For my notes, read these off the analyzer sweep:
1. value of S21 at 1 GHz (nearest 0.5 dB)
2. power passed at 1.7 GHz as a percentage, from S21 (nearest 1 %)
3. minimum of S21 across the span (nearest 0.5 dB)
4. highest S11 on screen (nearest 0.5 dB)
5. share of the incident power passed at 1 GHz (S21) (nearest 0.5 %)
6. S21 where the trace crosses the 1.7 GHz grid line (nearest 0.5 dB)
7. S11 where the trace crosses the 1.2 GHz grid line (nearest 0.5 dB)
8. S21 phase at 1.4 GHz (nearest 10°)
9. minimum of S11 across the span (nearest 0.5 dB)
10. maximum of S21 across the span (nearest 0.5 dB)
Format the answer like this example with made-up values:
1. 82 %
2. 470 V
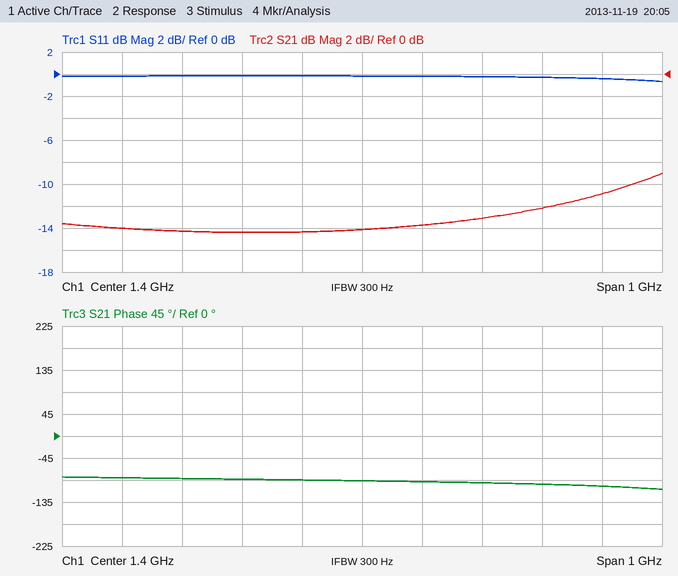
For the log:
1. -14.0 dB
2. 6 %
3. -14.5 dB
4. 0.0 dB
5. 4.0 %
6. -12.0 dB
7. 0.0 dB
8. -90°
9. -0.5 dB
10. -9.0 dB
